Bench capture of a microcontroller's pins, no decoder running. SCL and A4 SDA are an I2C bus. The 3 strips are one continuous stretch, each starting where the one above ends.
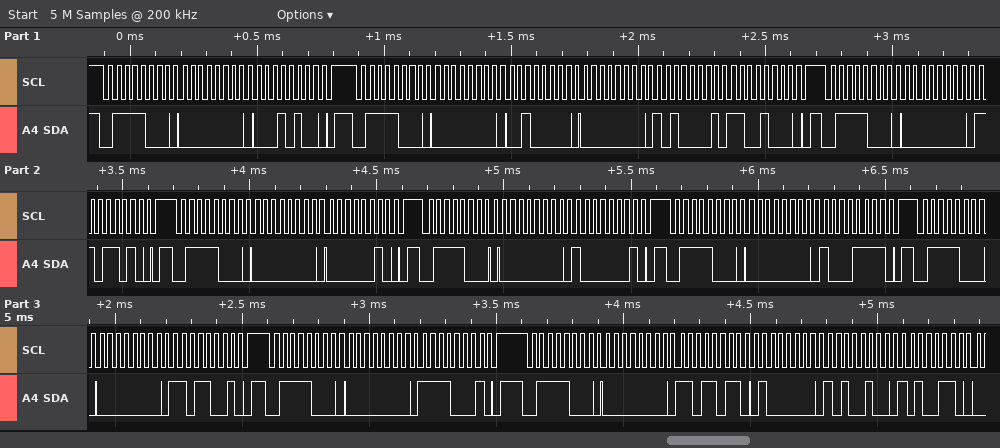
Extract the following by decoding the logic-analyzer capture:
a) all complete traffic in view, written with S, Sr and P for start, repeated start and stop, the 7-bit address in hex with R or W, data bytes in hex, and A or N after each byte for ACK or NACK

S 3CW A 00 A 14 A P S 3CW A 00 A 20 A 00 A A1 A C8 A P S 3CW A 00 A DA A P S 3CW A 00 A 02 A P S 3CW A 00 A 81 A P S 3CW A 00 A 8F A P S 3CW A 00 A D9 A P S 3CW A 00 A F1 A P S 3CW A 00 A DB A 40 A A4 A A6 A
